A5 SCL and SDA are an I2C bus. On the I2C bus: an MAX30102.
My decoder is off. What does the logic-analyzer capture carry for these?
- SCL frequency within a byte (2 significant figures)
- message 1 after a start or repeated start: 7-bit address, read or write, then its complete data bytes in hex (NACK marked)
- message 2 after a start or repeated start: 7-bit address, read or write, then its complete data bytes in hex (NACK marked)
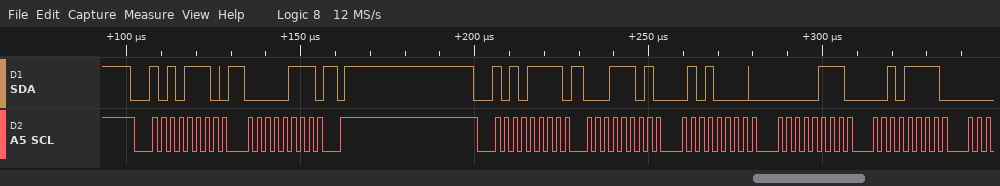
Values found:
400 kHz
0x57 write: 07
0x57 read: 1D 50 07 2F
